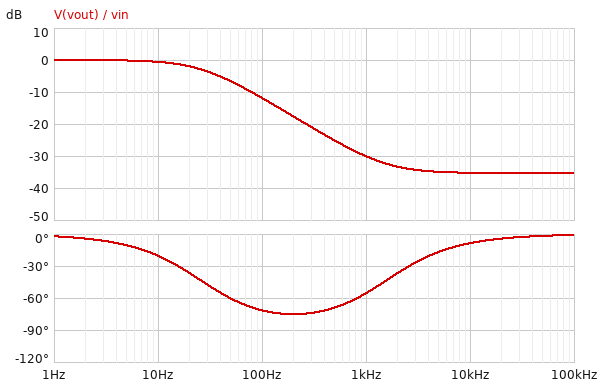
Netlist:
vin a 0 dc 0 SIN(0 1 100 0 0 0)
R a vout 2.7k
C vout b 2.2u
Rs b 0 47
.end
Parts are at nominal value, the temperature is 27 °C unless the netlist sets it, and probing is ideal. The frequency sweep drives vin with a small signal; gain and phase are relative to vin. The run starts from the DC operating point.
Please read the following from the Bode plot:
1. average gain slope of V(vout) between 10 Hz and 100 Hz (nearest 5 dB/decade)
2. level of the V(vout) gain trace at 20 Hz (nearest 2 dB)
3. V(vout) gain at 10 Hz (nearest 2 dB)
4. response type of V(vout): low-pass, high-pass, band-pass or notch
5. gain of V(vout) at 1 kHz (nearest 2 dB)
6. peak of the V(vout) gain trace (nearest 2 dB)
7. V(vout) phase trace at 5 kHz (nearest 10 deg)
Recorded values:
-10 dB/decade
-2 dB
0 dB
low-pass
-30 dB
0 dB
-20 deg
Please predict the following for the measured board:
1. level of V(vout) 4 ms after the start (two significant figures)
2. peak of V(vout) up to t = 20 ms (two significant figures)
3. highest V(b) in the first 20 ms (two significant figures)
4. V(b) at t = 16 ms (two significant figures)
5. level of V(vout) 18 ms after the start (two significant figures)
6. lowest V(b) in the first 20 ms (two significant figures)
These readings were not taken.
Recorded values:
370 mV
370 mV
16 mV
-13 mV
-140 mV
-18 mV
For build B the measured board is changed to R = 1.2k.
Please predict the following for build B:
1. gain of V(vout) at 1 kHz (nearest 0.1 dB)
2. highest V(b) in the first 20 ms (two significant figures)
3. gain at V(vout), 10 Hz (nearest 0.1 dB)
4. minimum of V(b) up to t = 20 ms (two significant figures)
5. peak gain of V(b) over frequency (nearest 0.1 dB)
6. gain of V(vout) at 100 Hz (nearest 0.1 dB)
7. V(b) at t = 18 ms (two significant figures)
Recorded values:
-23.2 dB
32 mV
-0.1 dB
-34 mV
-28.5 dB
-6.0 dB
-22 mV
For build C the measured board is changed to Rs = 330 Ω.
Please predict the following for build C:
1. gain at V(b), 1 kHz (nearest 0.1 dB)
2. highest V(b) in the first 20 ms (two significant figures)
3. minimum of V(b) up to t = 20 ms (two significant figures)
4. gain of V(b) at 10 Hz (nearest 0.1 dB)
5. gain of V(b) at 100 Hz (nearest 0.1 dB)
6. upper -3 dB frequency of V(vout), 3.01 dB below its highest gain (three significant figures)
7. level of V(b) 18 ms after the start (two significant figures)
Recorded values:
-19.3 dB
100 mV
-110 mV
-27.5 dB
-19.5 dB
24.2 Hz
-92 mV
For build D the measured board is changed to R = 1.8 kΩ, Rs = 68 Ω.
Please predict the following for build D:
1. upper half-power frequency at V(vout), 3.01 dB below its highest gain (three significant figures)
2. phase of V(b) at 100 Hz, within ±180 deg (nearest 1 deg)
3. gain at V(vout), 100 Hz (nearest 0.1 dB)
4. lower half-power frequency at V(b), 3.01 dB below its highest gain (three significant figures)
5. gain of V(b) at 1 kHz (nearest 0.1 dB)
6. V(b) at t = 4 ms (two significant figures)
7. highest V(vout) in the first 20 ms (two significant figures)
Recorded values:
38.8 Hz
21 deg
-8.8 dB
38.7 Hz
-28.8 dB
4.1 mV
480 mV
